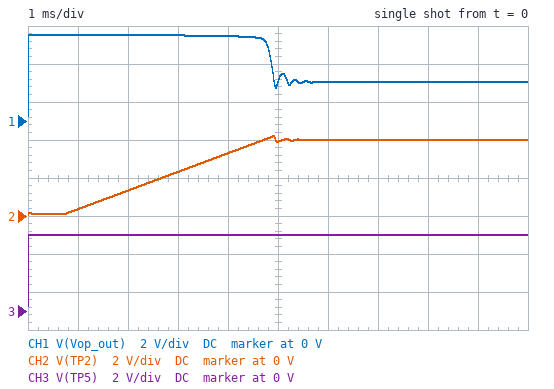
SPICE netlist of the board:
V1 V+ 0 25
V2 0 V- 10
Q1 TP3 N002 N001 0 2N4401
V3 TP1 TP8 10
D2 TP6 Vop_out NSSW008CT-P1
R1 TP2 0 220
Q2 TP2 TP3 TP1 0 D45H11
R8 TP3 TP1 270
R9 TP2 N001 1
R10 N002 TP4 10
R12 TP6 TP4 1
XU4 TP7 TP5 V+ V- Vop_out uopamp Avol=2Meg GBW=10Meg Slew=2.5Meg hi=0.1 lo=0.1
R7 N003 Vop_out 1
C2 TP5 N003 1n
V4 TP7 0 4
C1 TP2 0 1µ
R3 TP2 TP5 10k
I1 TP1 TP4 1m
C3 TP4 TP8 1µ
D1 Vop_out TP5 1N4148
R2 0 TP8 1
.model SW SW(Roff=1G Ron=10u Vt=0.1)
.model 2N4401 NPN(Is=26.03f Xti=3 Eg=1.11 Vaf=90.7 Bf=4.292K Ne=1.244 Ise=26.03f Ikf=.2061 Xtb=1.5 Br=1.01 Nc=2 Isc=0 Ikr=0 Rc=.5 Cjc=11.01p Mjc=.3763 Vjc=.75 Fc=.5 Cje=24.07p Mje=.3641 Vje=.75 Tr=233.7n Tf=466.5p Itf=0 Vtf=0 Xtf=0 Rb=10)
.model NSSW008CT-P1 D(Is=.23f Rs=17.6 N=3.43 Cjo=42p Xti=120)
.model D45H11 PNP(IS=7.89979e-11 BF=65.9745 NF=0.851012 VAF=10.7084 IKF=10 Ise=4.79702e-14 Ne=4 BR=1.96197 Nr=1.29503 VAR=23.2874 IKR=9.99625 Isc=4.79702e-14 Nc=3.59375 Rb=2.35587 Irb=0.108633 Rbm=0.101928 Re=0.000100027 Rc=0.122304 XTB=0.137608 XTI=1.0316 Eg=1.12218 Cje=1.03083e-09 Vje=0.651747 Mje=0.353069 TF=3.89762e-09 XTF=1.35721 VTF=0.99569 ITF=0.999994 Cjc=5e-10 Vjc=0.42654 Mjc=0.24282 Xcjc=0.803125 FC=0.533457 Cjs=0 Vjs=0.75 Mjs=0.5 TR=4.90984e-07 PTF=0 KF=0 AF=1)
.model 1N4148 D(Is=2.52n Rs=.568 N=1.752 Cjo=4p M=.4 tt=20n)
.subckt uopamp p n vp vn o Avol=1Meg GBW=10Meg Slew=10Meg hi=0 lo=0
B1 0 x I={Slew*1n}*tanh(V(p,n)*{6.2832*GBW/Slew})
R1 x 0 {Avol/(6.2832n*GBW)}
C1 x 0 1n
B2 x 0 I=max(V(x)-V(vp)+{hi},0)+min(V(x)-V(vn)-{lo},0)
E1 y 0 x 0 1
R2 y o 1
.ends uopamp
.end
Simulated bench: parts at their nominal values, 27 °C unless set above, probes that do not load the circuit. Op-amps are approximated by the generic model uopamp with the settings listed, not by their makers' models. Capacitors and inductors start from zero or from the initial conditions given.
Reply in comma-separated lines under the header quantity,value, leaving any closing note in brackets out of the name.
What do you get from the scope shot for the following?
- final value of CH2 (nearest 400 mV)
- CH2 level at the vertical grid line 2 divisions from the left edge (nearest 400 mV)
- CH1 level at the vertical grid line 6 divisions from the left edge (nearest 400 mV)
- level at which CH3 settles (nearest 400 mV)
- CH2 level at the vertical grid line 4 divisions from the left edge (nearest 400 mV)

quantity,value
final value of CH2,4.0 V
CH2 level at the vertical grid line 2 divisions from the left edge,1.2 V
CH1 level at the vertical grid line 6 divisions from the left edge,2.0 V
level at which CH3 settles,4.0 V
CH2 level at the vertical grid line 4 divisions from the left edge,3.2 V
